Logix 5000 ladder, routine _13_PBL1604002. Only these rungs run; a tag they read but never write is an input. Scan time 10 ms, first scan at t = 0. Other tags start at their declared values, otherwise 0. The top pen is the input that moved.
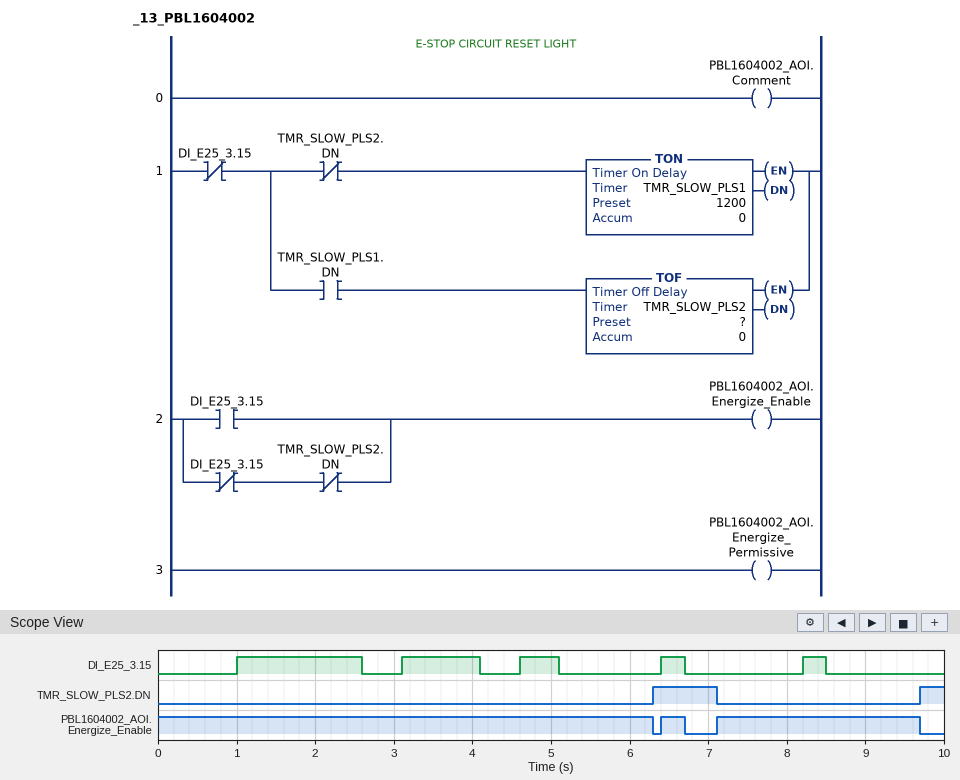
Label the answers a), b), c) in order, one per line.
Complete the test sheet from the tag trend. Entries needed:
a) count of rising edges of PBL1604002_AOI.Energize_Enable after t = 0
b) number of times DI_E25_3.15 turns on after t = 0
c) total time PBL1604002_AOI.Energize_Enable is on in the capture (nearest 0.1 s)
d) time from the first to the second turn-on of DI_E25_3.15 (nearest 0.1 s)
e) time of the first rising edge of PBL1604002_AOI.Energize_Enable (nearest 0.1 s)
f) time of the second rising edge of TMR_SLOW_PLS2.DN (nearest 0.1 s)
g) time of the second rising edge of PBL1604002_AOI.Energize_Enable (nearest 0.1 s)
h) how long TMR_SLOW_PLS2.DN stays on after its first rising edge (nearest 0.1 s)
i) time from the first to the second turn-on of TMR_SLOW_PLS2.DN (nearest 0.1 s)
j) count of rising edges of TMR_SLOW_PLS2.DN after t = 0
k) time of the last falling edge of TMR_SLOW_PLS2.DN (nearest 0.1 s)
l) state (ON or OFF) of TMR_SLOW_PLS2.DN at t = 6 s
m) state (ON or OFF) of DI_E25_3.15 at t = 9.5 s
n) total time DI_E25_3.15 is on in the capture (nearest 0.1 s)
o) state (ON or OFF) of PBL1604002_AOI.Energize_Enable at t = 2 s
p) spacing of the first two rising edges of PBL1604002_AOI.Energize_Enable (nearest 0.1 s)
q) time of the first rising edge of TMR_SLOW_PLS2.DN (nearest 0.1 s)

a) 2
b) 5
c) 9.2 s
d) 2.1 s
e) 6.4 s
f) 9.7 s
g) 7.1 s
h) 0.8 s
i) 3.4 s
j) 2
k) 7.1 s
l) OFF
m) OFF
n) 3.7 s
o) ON
p) 0.7 s
q) 6.3 s
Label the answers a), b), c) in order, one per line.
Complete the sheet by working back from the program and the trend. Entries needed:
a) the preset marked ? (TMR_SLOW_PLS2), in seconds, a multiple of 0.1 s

a) 0.8 s
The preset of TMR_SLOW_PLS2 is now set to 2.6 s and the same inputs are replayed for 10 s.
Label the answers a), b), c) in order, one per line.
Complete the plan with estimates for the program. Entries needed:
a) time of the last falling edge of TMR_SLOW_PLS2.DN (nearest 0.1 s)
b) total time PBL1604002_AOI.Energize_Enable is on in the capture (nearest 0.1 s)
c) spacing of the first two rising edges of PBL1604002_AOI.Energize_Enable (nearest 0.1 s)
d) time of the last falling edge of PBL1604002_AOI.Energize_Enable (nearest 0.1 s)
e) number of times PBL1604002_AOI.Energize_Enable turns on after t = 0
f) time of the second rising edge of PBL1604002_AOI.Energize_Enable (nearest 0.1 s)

a) 8.9 s
b) 8.0 s
c) 1.8 s
d) 8.5 s
e) 3
f) 8.2 s
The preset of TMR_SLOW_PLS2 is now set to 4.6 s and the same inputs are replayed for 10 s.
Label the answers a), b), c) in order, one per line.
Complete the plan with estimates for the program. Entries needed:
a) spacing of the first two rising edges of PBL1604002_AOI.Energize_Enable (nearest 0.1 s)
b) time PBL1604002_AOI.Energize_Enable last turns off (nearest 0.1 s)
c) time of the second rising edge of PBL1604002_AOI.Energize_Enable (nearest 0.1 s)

a) 1.8 s
b) 8.5 s
c) 8.2 s
